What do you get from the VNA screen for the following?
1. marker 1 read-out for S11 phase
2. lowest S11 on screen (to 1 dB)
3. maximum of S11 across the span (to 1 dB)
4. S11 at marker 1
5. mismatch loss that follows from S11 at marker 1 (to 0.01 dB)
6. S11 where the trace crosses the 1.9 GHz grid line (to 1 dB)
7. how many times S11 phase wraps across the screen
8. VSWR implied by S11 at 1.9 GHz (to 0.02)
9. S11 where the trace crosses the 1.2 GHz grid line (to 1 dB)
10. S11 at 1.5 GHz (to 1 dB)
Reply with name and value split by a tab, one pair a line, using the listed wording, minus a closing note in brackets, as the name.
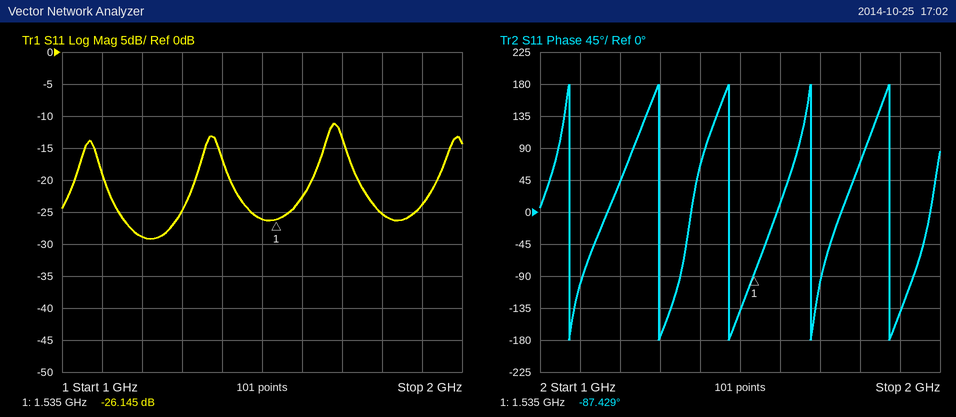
marker 1 read-out for S11 phase	-87.429°
lowest S11 on screen	-29 dB
maximum of S11 across the span	-11 dB
S11 at marker 1	-26.145 dB
mismatch loss that follows from S11 at marker 1	0.01 dB
S11 where the trace crosses the 1.9 GHz grid line	-24 dB
how many times S11 phase wraps across the screen	5
VSWR implied by S11 at 1.9 GHz	1.14
S11 where the trace crosses the 1.2 GHz grid line	-29 dB
S11 at 1.5 GHz	-26 dB
